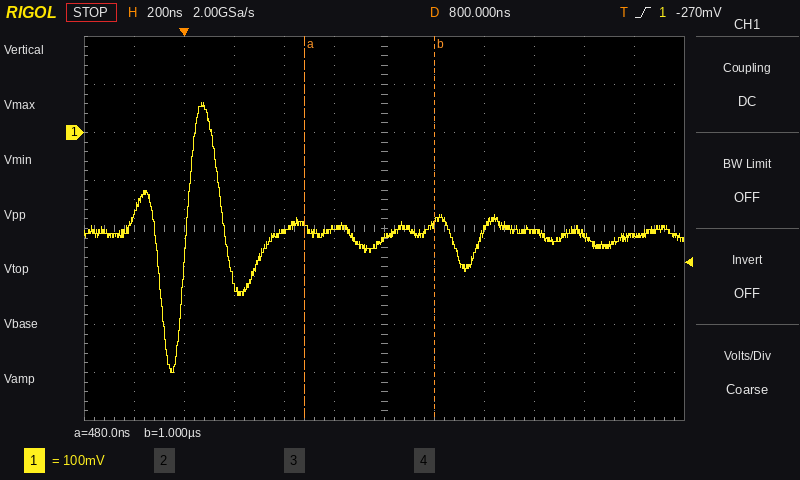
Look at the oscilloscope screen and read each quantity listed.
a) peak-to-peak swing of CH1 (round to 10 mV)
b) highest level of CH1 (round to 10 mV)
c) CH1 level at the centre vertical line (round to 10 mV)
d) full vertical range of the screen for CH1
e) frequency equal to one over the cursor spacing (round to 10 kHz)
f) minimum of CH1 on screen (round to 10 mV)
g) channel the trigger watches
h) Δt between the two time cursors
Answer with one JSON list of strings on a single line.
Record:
["560 mV", "60 mV", "-220 mV", "800 mV", "1.92 MHz", "-500 mV", "CH1", "520 ns"]
